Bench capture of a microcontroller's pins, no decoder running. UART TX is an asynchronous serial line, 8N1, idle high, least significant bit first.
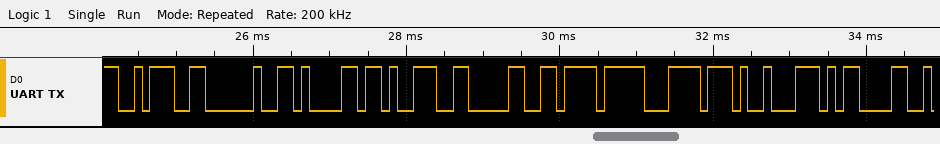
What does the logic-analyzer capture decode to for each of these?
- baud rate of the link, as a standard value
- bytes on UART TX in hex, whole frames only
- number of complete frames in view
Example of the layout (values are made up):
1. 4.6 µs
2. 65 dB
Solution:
1. 9600 baud
2. 0x3A 0x20 0x61 0x39 0x30 0xEF 0xBC 0x89 0x0D
3. 9
